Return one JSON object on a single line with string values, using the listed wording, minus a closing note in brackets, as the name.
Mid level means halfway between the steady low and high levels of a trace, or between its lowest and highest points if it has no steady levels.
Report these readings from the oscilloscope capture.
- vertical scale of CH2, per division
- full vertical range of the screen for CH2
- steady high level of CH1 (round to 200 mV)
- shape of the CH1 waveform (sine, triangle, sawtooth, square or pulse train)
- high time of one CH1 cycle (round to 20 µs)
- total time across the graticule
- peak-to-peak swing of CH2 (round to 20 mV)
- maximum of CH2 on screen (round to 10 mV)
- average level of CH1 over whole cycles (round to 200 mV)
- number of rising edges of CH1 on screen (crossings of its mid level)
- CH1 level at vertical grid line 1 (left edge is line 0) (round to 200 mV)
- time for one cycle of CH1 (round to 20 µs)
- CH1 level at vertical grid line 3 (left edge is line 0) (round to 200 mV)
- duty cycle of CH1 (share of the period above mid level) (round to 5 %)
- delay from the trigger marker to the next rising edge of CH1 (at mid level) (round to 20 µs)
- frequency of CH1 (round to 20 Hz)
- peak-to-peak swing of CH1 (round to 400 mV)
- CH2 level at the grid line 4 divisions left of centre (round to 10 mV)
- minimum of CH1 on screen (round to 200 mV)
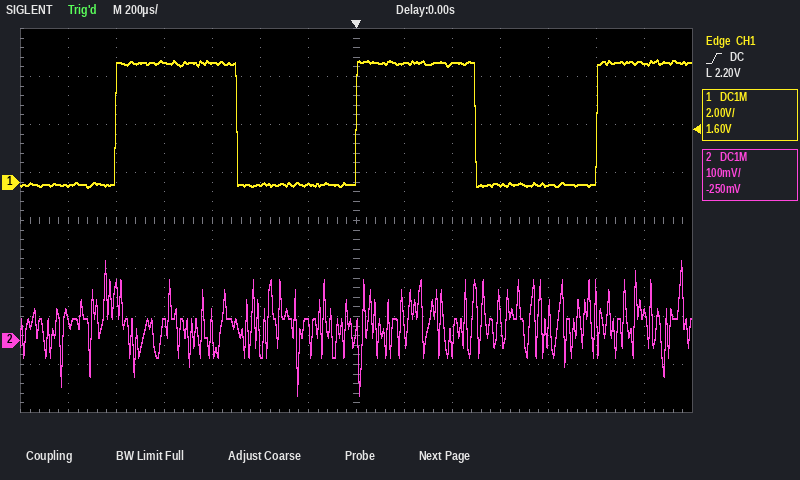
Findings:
{"vertical scale of CH2, per division": "100 mV", "full vertical range of the screen for CH2": "800 mV", "steady high level of CH1": "5.0 V", "shape of the CH1 waveform": "square", "high time of one CH1 cycle": "500 µs", "total time across the graticule": "2.8 ms", "peak-to-peak swing of CH2": "280 mV", "maximum of CH2 on screen": "170 mV", "average level of CH1 over whole cycles": "2.4 V", "number of rising edges of CH1 on screen": "3", "CH1 level at vertical grid line 1 (left edge is line 0)": "-200 mV", "time for one cycle of CH1": "1.00 ms", "CH1 level at vertical grid line 3 (left edge is line 0)": "5.0 V", "duty cycle of CH1 (share of the period above mid level)": "50 %", "delay from the trigger marker to the next rising edge of CH1 (at mid level)": "1.00 ms", "frequency of CH1": "1.00 kHz", "peak-to-peak swing of CH1": "5.2 V", "CH2 level at the grid line 4 divisions left of centre": "40 mV", "minimum of CH1 on screen": "-200 mV"}
